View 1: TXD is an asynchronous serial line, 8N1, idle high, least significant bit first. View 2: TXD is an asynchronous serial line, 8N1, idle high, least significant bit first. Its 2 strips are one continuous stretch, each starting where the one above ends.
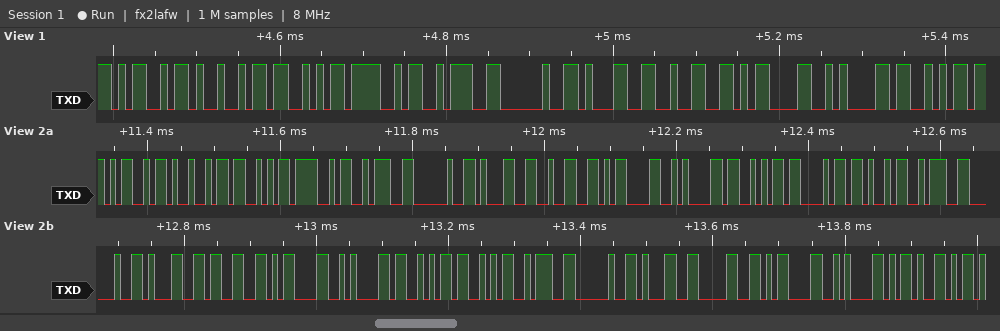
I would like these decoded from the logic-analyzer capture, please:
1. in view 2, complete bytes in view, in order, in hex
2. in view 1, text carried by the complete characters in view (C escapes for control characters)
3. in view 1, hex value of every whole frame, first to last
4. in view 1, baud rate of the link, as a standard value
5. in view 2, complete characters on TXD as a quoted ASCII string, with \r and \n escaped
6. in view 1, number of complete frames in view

4D 49 53 4F 3A 20 31 32 0D 0A 53 43 4B 3A 20 31 33 0D 0A 53 53 3A 20 31 30 0D 0A 2D
"MISO: 12\r\nS"
4D 49 53 4F 3A 20 31 32 0D 0A 53
115200 baud
"MISO: 12\r\nSCK: 13\r\nSS: 10\r\n-"
11
